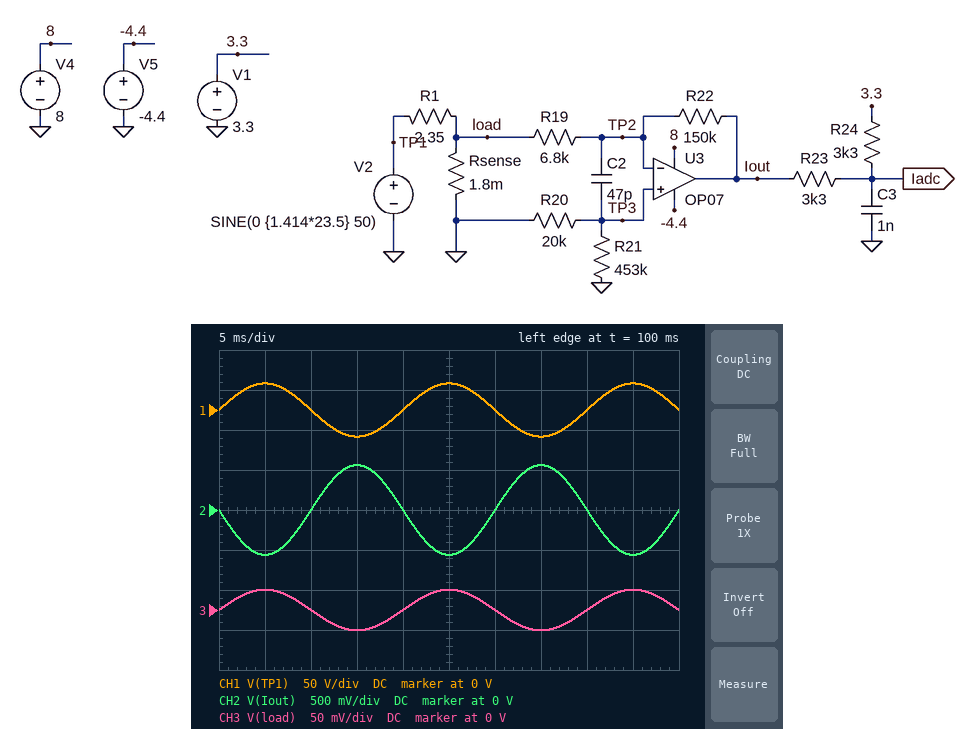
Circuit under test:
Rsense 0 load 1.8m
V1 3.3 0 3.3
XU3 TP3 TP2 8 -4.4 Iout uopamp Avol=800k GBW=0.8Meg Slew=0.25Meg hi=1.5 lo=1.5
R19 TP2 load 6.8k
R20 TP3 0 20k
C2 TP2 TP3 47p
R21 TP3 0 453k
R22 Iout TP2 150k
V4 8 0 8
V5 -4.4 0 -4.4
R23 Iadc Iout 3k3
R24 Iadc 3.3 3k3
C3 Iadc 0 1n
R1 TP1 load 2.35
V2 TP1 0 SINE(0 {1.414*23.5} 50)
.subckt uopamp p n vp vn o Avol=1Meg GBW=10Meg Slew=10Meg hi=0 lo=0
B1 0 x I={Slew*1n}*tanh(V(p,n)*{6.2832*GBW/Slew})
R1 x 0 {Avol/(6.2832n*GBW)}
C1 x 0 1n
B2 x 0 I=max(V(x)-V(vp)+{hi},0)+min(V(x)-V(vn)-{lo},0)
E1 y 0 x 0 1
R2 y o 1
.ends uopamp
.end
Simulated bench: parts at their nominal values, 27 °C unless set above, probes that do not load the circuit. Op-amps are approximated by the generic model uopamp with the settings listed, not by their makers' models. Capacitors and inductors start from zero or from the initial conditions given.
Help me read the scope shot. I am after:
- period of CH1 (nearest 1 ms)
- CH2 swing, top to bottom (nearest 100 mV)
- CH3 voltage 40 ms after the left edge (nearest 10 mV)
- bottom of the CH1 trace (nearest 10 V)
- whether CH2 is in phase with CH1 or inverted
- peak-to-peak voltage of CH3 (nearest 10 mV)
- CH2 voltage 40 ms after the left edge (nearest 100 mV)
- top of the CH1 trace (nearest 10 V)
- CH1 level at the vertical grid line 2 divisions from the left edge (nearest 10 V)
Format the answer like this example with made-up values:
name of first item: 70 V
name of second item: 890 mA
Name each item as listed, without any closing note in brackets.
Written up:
period of CH1: 20 ms
CH2 swing, top to bottom: 1.1 V
CH3 voltage 40 ms after the left edge: 0 V
bottom of the CH1 trace: -30 V
whether CH2 is in phase with CH1 or inverted: inverted
peak-to-peak voltage of CH3: 50 mV
CH2 voltage 40 ms after the left edge: 0 V
top of the CH1 trace: 30 V
CH1 level at the vertical grid line 2 divisions from the left edge: 0 V
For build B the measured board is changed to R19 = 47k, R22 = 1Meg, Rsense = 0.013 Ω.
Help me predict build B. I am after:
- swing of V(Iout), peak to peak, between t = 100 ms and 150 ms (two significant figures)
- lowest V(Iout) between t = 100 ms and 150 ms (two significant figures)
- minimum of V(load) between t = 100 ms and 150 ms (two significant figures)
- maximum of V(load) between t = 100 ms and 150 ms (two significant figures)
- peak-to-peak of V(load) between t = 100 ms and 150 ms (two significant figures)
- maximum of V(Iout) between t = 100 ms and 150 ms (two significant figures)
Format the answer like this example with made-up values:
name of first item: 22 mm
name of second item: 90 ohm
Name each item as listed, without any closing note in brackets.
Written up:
swing of V(Iout), peak to peak, between t = 100 ms and 150 ms: 6.8 V
lowest V(Iout) between t = 100 ms and 150 ms: -2.9 V
minimum of V(load) between t = 100 ms and 150 ms: -180 mV
maximum of V(load) between t = 100 ms and 150 ms: 180 mV
peak-to-peak of V(load) between t = 100 ms and 150 ms: 370 mV
maximum of V(Iout) between t = 100 ms and 150 ms: 3.9 V
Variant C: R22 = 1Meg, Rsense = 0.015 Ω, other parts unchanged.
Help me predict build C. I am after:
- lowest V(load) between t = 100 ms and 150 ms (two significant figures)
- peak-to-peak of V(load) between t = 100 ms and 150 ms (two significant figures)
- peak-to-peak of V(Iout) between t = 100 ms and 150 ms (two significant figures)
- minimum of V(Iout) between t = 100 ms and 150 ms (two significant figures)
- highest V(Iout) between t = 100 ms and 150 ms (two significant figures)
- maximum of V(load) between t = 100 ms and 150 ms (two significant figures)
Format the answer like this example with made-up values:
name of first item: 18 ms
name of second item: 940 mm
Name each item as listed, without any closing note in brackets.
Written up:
lowest V(load) between t = 100 ms and 150 ms: -210 mV
peak-to-peak of V(load) between t = 100 ms and 150 ms: 420 mV
peak-to-peak of V(Iout) between t = 100 ms and 150 ms: 9.4 V
minimum of V(Iout) between t = 100 ms and 150 ms: -2.9 V
highest V(Iout) between t = 100 ms and 150 ms: 6.5 V
maximum of V(load) between t = 100 ms and 150 ms: 210 mV
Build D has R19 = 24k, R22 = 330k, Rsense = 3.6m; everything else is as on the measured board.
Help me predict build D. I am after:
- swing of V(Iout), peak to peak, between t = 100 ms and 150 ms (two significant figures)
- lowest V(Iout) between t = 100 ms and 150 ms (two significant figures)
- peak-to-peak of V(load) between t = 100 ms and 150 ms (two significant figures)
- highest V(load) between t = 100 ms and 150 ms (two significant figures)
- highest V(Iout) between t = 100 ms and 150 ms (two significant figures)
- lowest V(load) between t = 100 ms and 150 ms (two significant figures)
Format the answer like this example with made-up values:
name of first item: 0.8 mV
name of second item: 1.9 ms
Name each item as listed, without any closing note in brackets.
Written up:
swing of V(Iout), peak to peak, between t = 100 ms and 150 ms: 1.4 V
lowest V(Iout) between t = 100 ms and 150 ms: -700 mV
peak-to-peak of V(load) between t = 100 ms and 150 ms: 100 mV
highest V(load) between t = 100 ms and 150 ms: 51 mV
highest V(Iout) between t = 100 ms and 150 ms: 700 mV
lowest V(load) between t = 100 ms and 150 ms: -51 mV
